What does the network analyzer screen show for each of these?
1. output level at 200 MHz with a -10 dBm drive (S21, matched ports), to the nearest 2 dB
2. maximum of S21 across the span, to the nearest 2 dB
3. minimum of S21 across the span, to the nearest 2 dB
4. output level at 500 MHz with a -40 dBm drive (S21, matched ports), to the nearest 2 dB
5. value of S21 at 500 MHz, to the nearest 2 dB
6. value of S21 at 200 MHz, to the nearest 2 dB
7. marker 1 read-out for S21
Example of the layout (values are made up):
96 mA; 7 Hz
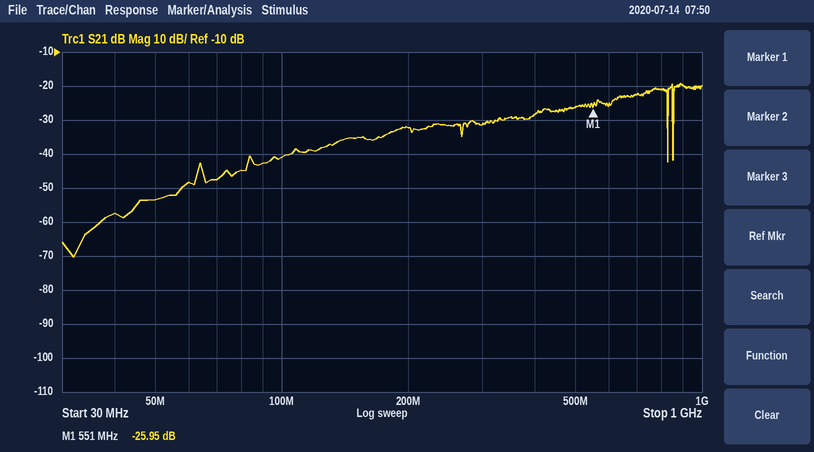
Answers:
-42 dBm; -20 dB; -70 dB; -66 dBm; -26 dB; -32 dB; -25.95 dB
